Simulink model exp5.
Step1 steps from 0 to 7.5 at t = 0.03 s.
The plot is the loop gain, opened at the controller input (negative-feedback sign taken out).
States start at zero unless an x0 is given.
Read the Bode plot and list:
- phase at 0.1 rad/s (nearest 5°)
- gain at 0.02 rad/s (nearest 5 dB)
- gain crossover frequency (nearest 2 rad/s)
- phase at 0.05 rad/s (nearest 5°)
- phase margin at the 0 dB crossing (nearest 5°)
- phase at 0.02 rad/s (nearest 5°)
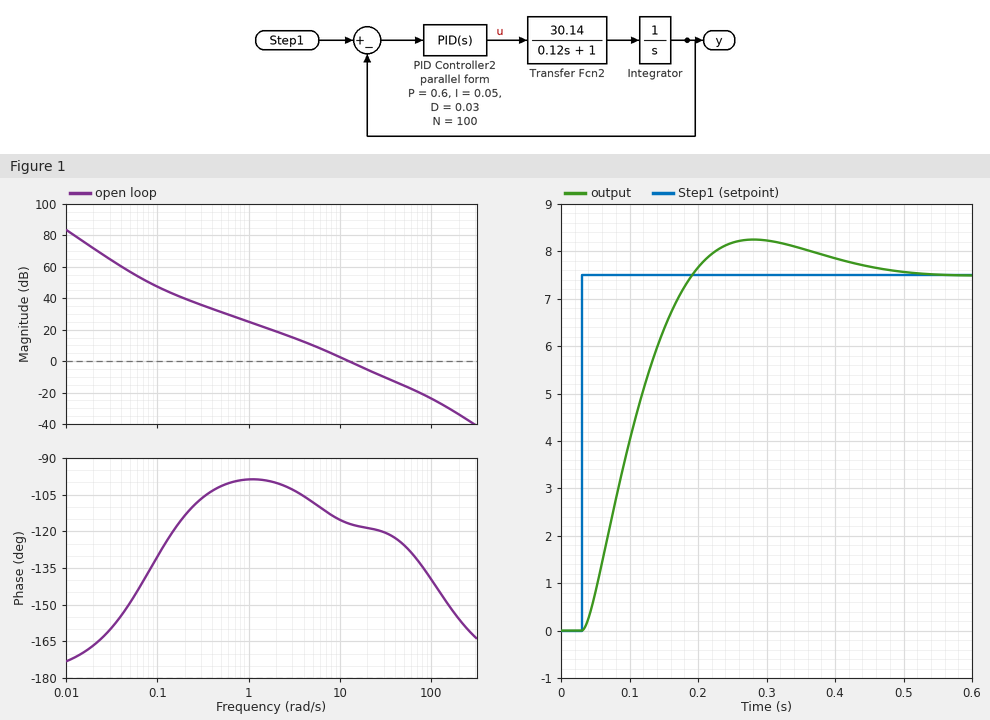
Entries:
-130°
70 dB
12 rad/s
-150°
65°
-165°
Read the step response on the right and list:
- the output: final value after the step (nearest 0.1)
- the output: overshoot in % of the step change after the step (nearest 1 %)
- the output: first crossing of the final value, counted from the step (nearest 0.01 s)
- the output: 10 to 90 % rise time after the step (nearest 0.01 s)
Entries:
7.5
10 %
0.16 s
0.11 s
